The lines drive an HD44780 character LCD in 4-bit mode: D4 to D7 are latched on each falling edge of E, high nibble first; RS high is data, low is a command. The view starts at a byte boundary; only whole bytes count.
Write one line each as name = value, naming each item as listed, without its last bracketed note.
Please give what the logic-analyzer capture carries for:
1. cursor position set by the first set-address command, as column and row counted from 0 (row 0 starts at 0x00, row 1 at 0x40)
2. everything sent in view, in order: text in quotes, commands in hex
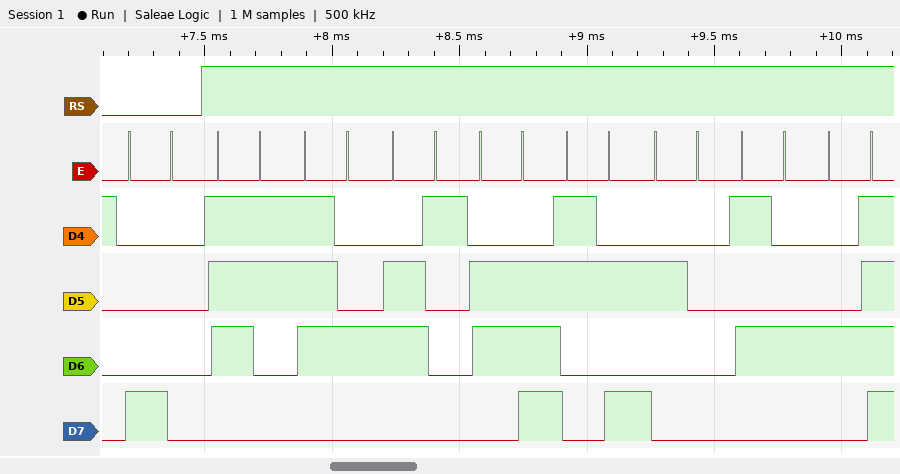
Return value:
cursor position set by the first set-address command, as column and row counted from 0 = column 0, row 0
everything sent in view, in order: text in quotes, commands in hex = 0x80 "stan: TO"
